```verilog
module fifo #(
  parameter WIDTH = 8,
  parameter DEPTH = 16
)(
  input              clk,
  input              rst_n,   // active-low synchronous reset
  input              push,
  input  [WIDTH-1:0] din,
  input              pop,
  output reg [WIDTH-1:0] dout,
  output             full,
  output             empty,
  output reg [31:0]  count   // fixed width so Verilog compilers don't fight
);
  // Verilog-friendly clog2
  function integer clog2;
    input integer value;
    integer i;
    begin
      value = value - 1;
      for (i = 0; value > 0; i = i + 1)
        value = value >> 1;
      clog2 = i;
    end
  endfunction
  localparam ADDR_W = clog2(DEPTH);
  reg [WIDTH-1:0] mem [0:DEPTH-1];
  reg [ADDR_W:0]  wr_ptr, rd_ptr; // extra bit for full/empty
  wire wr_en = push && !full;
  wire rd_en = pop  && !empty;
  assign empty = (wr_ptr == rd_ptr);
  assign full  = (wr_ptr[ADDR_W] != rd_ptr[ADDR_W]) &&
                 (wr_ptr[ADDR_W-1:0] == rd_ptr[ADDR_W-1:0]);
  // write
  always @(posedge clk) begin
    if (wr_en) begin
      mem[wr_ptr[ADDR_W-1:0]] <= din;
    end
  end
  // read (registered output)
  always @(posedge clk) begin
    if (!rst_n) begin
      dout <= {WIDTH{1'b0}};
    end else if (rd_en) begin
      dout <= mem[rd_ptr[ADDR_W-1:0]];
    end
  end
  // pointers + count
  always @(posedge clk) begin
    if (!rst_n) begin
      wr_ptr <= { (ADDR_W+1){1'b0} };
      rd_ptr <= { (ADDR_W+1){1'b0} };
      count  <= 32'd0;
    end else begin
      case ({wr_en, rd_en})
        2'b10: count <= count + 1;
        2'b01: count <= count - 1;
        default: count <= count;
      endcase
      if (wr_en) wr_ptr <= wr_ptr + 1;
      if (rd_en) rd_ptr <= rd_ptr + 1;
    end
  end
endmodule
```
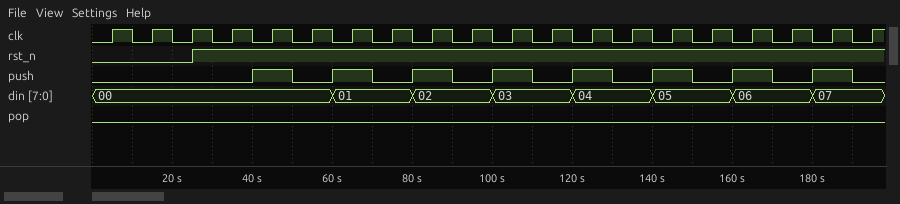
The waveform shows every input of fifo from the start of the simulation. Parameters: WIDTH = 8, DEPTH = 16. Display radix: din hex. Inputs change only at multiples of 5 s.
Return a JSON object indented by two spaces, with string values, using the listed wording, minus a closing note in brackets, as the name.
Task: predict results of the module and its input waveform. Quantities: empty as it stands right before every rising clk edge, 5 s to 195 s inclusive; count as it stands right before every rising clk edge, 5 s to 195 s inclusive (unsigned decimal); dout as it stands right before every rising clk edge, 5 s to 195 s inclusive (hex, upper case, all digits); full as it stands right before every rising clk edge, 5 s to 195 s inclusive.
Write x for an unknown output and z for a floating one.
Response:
{
  "empty as it stands right before every rising clk edge, 5 s to 195 s inclusive": "x 1 1 1 1 0 0 0 0 0 0 0 0 0 0 0 0 0 0 0",
  "count as it stands right before every rising clk edge, 5 s to 195 s inclusive": "x, 0, 0, 0, 0, 1, 1, 2, 2, 3, 3, 4, 4, 5, 5, 6, 6, 7, 7, 8",
  "dout as it stands right before every rising clk edge, 5 s to 195 s inclusive": "x, 00, 00, 00, 00, 00, 00, 00, 00, 00, 00, 00, 00, 00, 00, 00, 00, 00, 00, 00",
  "full as it stands right before every rising clk edge, 5 s to 195 s inclusive": "x 0 0 0 0 0 0 0 0 0 0 0 0 0 0 0 0 0 0 0"
}
